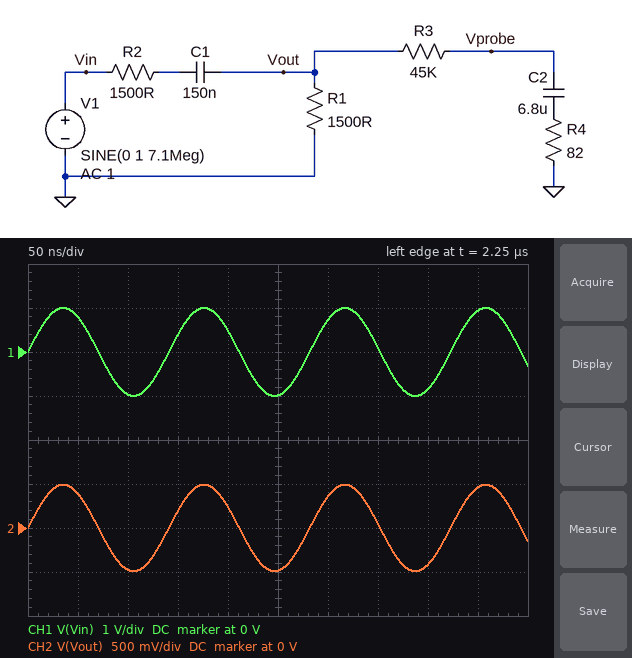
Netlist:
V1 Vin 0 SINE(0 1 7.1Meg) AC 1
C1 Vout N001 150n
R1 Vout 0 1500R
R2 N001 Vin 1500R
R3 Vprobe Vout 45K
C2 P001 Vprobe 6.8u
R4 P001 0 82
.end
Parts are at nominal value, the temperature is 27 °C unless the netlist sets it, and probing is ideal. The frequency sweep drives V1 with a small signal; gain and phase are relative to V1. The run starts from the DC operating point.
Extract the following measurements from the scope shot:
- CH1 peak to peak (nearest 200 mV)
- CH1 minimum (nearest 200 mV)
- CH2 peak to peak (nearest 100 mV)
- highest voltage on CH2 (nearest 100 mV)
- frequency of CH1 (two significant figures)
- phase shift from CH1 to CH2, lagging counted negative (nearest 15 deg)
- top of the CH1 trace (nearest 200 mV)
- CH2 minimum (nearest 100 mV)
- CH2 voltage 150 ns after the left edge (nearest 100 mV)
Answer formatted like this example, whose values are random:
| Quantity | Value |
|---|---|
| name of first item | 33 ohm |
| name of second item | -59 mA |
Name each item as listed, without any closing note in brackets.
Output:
| Quantity | Value |
|---|---|
| CH1 peak to peak | 2.0 V |
| CH1 minimum | -1.0 V |
| CH2 peak to peak | 1.0 V |
| highest voltage on CH2 | 500 mV |
| frequency of CH1 | 7.1 MHz |
| phase shift from CH1 to CH2, lagging counted negative | 0 deg |
| top of the CH1 trace | 1.0 V |
| CH2 minimum | -500 mV |
| CH2 voltage 150 ns after the left edge | 200 mV |
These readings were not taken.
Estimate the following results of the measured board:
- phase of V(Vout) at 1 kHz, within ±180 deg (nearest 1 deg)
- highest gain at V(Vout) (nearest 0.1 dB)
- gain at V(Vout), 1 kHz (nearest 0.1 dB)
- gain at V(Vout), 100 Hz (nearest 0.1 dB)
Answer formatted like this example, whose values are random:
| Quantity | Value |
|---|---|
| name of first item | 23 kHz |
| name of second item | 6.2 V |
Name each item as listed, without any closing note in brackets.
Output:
| Quantity | Value |
|---|---|
| phase of V(Vout) at 1 kHz, within ±180 deg | 20 deg |
| highest gain at V(Vout) | -6.2 dB |
| gain at V(Vout), 1 kHz | -6.7 dB |
| gain at V(Vout), 100 Hz | -17.6 dB |
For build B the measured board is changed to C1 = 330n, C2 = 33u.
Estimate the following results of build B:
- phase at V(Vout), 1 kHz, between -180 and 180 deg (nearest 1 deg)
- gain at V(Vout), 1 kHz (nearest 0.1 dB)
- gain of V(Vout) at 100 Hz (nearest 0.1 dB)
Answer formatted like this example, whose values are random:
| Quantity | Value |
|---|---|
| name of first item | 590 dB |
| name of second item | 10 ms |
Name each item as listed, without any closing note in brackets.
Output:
| Quantity | Value |
|---|---|
| phase at V(Vout), 1 kHz, between -180 and 180 deg | 9 deg |
| gain at V(Vout), 1 kHz | -6.3 dB |
| gain of V(Vout) at 100 Hz | -11.8 dB |
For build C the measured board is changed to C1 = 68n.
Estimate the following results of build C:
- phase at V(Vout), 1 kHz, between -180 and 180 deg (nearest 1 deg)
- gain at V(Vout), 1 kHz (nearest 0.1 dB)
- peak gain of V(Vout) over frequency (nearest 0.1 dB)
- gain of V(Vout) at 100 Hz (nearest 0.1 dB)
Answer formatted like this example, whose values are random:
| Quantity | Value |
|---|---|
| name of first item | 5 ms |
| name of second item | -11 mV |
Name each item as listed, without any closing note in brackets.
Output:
| Quantity | Value |
|---|---|
| phase at V(Vout), 1 kHz, between -180 and 180 deg | 38 deg |
| gain at V(Vout), 1 kHz | -8.3 dB |
| peak gain of V(Vout) over frequency | -6.2 dB |
| gain of V(Vout) at 100 Hz | -24.2 dB |
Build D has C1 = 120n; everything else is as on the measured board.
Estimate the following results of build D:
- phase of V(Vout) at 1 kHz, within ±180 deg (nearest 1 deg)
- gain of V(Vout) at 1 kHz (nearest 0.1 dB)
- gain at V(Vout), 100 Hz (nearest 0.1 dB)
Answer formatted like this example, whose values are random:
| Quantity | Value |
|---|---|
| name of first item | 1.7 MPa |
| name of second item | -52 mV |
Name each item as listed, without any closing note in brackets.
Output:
| Quantity | Value |
|---|---|
| phase of V(Vout) at 1 kHz, within ±180 deg | 24 deg |
| gain of V(Vout) at 1 kHz | -7.0 dB |
| gain at V(Vout), 100 Hz | -19.4 dB |
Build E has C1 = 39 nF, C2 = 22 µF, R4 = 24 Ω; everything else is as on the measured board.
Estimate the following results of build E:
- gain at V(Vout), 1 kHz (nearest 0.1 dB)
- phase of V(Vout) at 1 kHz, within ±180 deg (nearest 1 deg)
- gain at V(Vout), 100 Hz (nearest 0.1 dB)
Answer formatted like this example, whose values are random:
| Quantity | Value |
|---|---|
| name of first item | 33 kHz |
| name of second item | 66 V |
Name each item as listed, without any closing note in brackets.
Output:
| Quantity | Value |
|---|---|
| gain at V(Vout), 1 kHz | -10.8 dB |
| phase of V(Vout) at 1 kHz, within ±180 deg | 54 deg |
| gain at V(Vout), 100 Hz | -29.0 dB |
